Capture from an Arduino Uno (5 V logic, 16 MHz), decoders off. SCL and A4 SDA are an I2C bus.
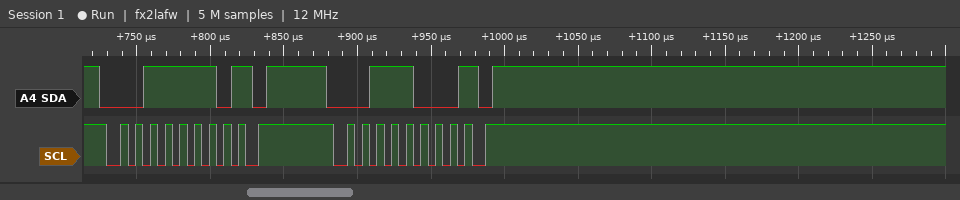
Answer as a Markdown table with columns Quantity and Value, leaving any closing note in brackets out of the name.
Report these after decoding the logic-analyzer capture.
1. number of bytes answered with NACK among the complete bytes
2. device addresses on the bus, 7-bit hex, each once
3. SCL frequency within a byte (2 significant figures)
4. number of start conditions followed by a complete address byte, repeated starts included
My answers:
| Quantity | Value |
|---|---|
| number of bytes answered with NACK among the complete bytes | 2 |
| device addresses on the bus, 7-bit hex, each once | 0x1F 0x1C |
| SCL frequency within a byte | 100 kHz |
| number of start conditions followed by a complete address byte, repeated starts included | 2 |
